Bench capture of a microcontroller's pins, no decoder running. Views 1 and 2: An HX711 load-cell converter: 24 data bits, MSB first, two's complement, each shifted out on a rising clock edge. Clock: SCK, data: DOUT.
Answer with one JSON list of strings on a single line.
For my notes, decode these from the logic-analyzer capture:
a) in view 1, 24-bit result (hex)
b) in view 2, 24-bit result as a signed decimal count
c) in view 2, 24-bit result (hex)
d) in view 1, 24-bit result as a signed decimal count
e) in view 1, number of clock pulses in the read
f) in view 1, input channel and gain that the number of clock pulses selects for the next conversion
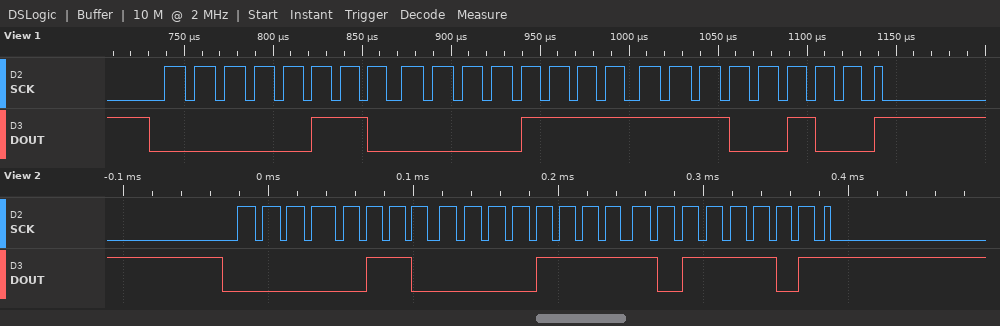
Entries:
["0x060FE4", "397245", "0x060FBD", "397284", "25", "channel A, gain 128"]
